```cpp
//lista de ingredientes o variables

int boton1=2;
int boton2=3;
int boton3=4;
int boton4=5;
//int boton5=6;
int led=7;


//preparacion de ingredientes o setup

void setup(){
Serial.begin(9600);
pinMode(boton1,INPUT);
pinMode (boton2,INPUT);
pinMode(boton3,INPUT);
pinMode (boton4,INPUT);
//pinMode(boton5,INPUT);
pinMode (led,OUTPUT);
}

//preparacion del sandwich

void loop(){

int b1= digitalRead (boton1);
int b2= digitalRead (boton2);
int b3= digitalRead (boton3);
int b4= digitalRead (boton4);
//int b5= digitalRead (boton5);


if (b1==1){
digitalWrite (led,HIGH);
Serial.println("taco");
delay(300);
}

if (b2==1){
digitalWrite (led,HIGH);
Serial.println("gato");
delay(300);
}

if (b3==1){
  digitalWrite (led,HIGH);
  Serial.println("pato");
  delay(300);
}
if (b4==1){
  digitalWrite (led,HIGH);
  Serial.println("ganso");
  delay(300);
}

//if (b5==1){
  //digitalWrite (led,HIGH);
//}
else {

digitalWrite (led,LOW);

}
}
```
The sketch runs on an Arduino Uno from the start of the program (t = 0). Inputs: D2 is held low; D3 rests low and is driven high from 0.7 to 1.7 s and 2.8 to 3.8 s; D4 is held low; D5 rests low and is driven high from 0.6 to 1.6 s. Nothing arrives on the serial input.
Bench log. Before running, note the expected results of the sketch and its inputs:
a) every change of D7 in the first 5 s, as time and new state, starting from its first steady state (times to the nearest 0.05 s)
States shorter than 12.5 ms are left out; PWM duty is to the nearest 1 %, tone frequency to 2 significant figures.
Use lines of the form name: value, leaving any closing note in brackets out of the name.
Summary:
every change of D7 in the first 5 s, as time and new state, starting from its first steady state: 0 s low; 0.6 s high; 2.1 s low; 2.8 s high; 4 s low
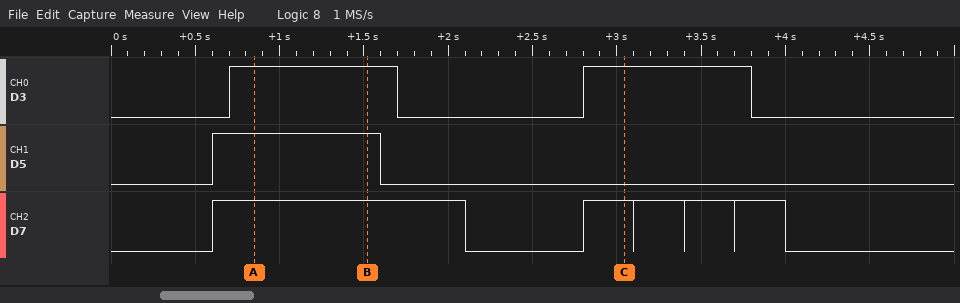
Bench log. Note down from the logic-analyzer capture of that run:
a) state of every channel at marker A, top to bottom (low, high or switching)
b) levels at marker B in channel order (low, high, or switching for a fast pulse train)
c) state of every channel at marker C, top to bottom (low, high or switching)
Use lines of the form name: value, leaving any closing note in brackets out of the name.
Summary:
state of every channel at marker A, top to bottom: D3 high, D5 high, D7 high
levels at marker B in channel order: D3 high, D5 high, D7 high
state of every channel at marker C, top to bottom: D3 high, D5 low, D7 high
